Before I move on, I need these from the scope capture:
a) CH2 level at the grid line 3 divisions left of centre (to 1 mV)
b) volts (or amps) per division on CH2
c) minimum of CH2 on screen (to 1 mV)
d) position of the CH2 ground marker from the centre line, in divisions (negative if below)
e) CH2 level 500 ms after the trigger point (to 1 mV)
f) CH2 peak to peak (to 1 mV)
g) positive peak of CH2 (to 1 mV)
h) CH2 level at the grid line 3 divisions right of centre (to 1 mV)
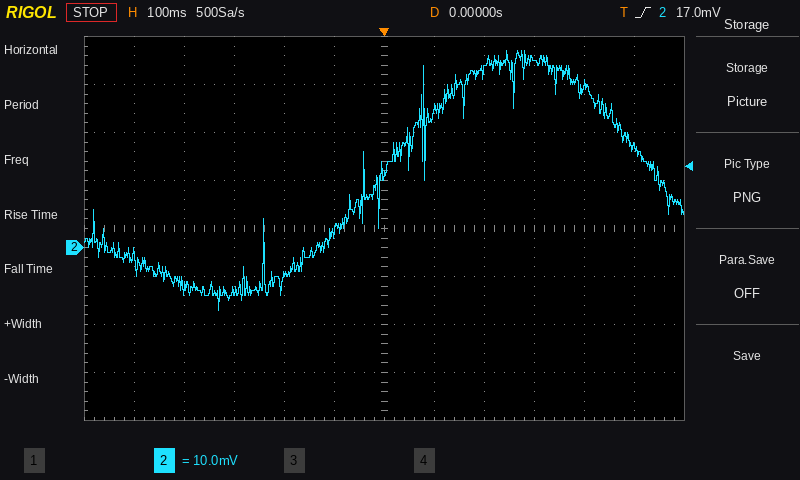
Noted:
-9 mV
10 mV
-13 mV
-0.4 div
21 mV
54 mV
41 mV
39 mV
